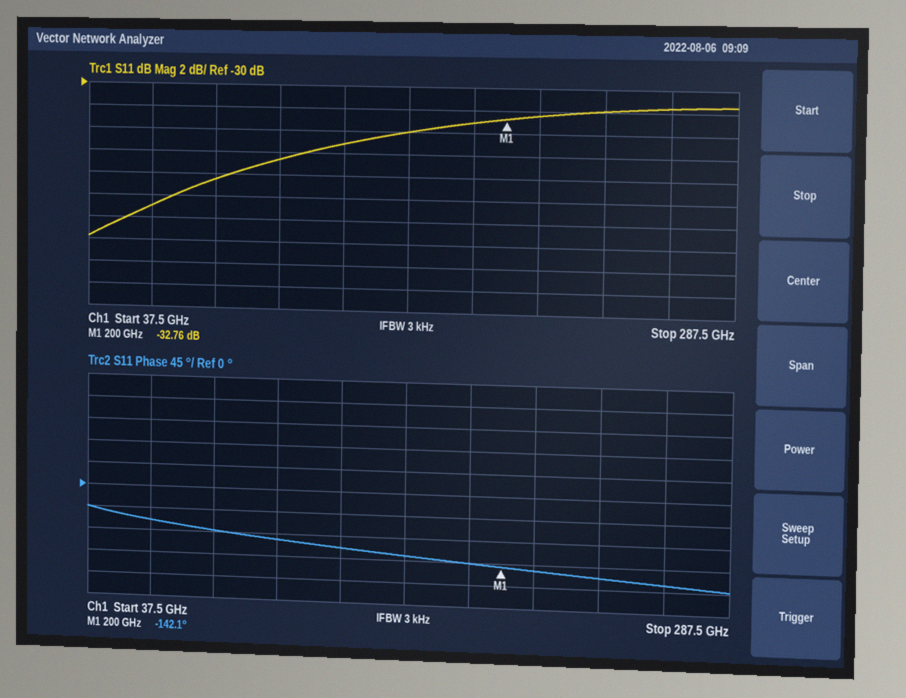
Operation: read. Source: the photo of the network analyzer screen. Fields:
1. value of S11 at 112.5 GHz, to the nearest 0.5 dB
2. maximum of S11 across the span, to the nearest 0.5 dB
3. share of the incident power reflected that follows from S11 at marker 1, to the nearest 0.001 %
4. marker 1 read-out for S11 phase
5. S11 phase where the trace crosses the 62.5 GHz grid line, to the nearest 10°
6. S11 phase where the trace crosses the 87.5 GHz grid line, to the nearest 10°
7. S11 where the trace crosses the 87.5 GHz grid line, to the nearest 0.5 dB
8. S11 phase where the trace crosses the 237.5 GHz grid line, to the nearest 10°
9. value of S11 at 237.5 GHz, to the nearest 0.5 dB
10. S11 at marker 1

-36.5 dB
-31.5 dB
0.053 %
-142.1°
-70°
-90°
-38.5 dB
-160°
-32.0 dB
-32.76 dB
